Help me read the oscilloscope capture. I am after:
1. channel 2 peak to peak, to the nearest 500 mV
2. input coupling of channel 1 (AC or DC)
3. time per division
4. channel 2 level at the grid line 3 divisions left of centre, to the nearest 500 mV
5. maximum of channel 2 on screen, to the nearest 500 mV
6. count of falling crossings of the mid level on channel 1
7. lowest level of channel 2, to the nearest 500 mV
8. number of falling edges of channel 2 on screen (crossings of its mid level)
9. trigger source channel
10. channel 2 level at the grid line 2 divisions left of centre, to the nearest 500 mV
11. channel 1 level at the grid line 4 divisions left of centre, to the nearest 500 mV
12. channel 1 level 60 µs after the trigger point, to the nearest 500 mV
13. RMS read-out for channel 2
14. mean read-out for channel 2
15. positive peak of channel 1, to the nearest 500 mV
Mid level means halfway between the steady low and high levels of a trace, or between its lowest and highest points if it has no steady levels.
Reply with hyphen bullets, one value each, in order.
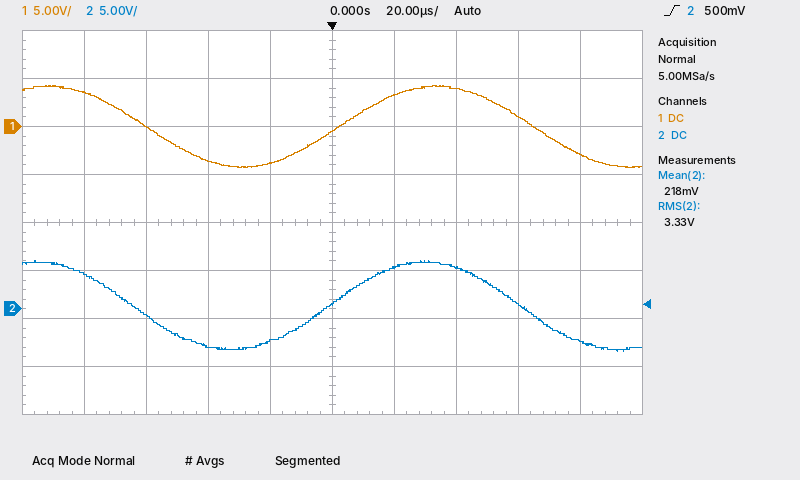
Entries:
- 9.5 V
- DC
- 20 µs
- -500 mV
- 5.0 V
- 2
- -4.5 V
- 2
- channel 2
- -4.0 V
- 3.5 V
- 1.0 V
- 3.33 V
- 218 mV
- 4.5 V
